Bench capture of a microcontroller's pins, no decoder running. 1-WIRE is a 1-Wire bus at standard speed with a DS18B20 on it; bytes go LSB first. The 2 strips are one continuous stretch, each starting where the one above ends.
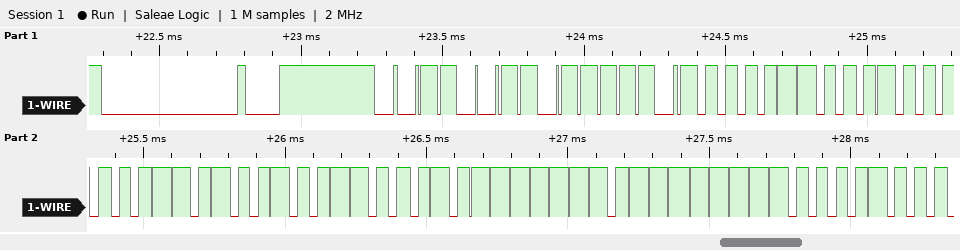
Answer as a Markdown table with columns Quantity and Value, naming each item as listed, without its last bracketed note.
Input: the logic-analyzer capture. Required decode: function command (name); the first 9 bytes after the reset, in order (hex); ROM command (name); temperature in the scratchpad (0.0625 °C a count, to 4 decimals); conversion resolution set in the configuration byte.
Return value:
| Quantity | Value |
|---|---|
| function command | Read Scratchpad |
| the first 9 bytes after the reset, in order | CC BE 30 02 4B 46 7F FF 10 |
| ROM command | Skip ROM |
| temperature in the scratchpad | 35.0000 °C |
| conversion resolution set in the configuration byte | 12 bits |
